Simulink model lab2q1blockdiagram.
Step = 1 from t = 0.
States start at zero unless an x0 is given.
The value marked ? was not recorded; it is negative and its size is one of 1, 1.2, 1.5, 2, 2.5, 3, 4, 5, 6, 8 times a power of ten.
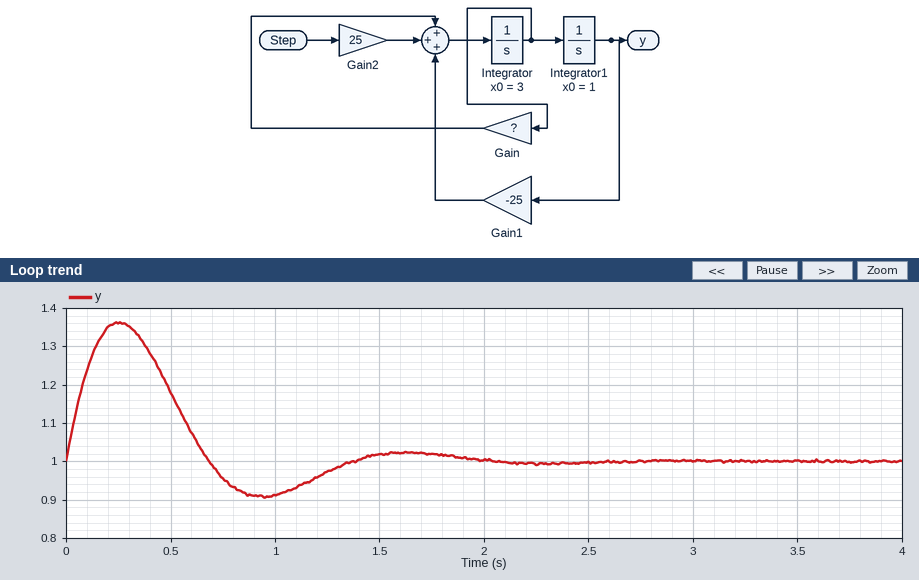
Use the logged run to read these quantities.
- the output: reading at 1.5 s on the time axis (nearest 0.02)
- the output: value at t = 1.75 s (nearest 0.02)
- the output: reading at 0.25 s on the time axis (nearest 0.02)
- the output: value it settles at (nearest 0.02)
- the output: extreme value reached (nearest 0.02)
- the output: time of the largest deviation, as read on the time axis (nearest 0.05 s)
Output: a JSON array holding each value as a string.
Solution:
["1.02", "1.02", "1.36", "1.00", "1.36", "0.25 s"]
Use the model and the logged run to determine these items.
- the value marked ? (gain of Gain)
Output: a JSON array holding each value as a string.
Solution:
["-4"]
